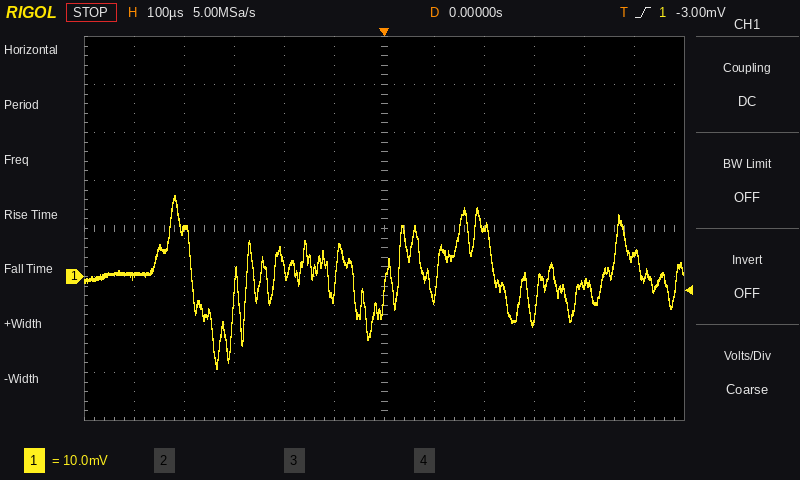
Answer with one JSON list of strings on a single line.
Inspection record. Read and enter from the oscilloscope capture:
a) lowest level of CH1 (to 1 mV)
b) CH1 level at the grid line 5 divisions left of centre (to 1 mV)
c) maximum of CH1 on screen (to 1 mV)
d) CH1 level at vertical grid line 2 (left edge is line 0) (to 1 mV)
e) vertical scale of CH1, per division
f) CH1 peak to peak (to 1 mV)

["-19 mV", "0 mV", "17 mV", "10 mV", "10 mV", "36 mV"]
